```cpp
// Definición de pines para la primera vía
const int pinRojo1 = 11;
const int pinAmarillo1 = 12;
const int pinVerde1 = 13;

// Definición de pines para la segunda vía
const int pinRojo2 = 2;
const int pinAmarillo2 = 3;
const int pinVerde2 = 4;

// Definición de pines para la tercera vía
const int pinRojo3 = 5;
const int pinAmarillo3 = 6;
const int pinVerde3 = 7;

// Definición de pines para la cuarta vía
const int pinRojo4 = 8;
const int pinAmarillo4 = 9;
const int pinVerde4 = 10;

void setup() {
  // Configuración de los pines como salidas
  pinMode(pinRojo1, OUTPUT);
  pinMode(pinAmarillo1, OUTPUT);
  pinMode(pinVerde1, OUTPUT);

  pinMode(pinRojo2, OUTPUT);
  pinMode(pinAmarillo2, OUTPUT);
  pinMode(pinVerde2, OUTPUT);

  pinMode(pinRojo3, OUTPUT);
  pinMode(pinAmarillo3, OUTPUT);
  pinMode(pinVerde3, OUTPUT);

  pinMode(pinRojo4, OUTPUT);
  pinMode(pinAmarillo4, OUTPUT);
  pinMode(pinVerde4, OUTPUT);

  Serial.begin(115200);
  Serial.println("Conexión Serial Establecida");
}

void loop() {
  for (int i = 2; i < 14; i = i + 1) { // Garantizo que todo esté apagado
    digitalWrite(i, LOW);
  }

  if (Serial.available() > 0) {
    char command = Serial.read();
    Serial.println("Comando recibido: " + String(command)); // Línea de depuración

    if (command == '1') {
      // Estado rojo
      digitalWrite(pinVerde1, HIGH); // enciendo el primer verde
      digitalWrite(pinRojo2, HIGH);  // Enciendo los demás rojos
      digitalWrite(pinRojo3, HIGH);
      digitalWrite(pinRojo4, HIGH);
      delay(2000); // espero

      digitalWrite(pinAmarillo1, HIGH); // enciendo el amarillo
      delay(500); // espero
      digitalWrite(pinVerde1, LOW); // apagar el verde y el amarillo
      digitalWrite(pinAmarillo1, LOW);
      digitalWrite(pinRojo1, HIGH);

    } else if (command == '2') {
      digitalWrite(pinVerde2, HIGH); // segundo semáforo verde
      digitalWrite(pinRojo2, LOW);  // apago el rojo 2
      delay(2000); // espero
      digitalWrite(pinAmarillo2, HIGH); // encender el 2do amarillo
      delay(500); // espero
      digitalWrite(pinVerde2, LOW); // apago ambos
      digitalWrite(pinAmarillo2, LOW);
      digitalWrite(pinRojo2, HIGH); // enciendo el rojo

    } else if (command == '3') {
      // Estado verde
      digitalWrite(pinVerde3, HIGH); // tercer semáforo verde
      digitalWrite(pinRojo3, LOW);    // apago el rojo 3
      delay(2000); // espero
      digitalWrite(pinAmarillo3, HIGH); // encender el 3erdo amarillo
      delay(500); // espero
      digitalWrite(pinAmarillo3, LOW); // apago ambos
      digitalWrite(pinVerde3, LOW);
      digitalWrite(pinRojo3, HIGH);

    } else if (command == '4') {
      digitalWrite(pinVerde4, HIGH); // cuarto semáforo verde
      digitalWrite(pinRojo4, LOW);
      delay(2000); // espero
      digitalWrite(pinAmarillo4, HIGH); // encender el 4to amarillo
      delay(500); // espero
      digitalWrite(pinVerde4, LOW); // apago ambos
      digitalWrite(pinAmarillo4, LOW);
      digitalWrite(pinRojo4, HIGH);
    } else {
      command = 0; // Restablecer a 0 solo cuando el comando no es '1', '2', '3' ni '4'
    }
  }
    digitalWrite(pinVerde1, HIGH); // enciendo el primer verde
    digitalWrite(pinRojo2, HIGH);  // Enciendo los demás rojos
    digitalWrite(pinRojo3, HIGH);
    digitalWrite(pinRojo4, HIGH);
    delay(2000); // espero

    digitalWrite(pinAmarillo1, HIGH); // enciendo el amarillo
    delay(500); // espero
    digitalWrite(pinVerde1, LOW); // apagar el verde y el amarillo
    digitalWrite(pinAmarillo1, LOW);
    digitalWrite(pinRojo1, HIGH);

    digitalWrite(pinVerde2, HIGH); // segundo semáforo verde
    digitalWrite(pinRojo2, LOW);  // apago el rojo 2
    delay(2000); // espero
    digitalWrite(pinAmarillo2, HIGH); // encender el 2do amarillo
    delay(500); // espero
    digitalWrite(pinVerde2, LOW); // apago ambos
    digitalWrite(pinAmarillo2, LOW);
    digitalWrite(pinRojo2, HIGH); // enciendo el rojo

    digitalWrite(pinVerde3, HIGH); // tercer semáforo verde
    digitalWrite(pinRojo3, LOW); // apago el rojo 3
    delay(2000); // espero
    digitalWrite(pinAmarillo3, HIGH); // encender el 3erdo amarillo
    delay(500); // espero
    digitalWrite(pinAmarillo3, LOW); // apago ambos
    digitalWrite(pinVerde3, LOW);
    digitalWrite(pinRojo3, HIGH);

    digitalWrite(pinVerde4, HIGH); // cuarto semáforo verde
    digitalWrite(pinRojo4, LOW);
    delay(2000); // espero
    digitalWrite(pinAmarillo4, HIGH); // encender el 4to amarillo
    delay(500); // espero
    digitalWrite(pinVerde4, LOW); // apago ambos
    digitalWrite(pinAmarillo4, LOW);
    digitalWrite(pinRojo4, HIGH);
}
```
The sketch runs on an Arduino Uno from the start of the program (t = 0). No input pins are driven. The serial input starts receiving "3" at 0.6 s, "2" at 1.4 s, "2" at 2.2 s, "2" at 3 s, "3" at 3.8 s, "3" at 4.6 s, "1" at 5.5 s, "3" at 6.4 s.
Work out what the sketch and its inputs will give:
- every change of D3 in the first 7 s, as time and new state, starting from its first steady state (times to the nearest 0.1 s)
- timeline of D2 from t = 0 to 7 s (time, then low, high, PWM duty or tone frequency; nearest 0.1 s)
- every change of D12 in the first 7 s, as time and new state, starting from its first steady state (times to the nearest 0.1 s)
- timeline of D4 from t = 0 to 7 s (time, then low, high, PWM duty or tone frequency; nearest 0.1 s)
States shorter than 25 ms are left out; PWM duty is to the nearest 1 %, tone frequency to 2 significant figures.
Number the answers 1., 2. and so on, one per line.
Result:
1. 0 s low; 4.5 s high; 5 s low
2. 0 s high; 2.5 s low; 5 s high
3. 0 s low; 2 s high; 2.5 s low
4. 0 s low; 2.5 s high; 5 s low
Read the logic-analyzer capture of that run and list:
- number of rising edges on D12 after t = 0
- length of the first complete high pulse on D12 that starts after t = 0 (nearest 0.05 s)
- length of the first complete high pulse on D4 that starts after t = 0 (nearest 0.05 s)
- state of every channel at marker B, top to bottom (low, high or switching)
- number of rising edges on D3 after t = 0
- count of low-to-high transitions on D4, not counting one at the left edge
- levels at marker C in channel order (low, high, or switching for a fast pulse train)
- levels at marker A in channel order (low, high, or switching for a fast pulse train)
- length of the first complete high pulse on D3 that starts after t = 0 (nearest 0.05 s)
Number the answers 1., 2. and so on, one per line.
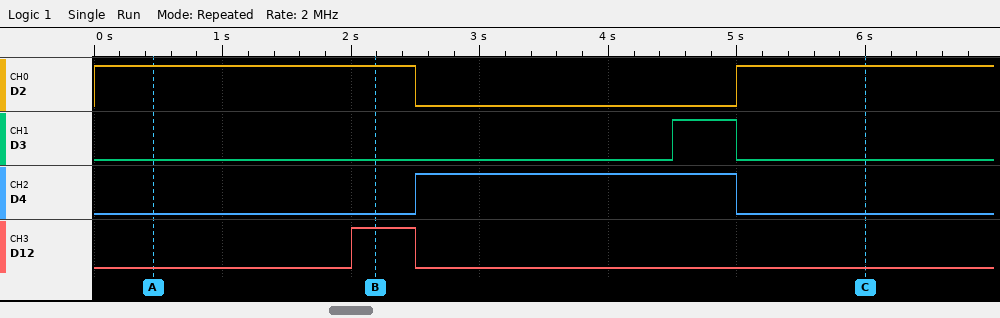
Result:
1. 1
2. 0.50 s
3. 2.50 s
4. D2 high, D3 low, D4 low, D12 high
5. 1
6. 1
7. D2 high, D3 low, D4 low, D12 low
8. D2 high, D3 low, D4 low, D12 low
9. 0.50 s
